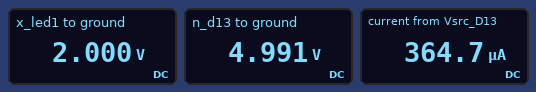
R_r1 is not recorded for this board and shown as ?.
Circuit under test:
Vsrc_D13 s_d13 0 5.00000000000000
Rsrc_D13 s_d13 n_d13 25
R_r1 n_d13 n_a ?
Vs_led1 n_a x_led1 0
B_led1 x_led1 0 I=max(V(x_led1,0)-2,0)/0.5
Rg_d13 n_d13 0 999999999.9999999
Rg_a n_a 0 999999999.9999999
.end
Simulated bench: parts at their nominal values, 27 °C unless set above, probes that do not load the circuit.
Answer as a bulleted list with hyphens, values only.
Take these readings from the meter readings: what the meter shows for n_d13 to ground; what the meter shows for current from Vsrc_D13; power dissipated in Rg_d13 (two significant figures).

- 4.991 V
- 364.7 µA
- 25 nW
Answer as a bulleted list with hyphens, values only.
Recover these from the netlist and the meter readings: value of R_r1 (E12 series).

- 8.2 kΩ
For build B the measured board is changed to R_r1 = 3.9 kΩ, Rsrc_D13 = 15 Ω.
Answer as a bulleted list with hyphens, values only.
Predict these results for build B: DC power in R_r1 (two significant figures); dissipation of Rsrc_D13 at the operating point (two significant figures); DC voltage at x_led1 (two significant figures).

- 2.3 mW
- 8.8 µW
- 2.0 V
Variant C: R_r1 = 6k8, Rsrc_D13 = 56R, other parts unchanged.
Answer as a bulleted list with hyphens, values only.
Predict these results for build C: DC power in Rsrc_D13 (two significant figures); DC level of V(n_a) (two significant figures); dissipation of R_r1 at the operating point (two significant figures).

- 11 µW
- 2.0 V
- 1.3 mW
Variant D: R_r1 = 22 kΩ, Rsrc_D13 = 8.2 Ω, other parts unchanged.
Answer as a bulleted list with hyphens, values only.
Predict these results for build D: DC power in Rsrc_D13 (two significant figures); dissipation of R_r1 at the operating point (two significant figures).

- 150 nW
- 410 µW
